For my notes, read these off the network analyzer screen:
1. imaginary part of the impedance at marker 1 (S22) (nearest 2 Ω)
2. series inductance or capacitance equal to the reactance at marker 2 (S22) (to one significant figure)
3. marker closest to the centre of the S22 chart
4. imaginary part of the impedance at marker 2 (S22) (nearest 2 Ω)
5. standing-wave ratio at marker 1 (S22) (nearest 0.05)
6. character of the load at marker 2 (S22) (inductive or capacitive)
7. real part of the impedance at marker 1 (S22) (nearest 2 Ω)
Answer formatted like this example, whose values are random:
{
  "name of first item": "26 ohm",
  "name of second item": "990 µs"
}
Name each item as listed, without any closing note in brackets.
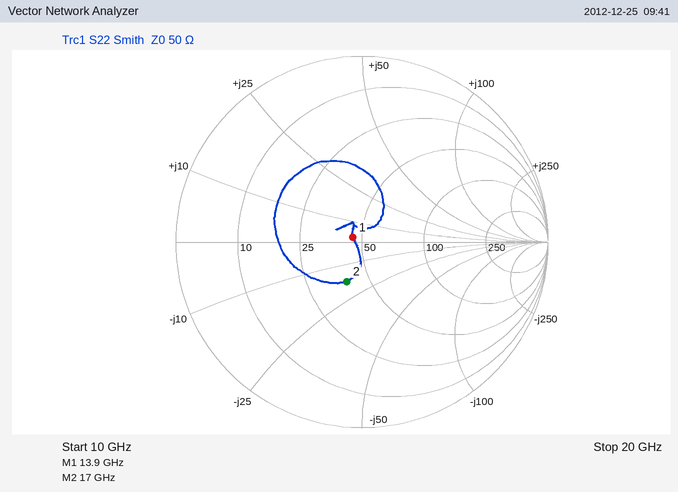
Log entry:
{
  "imaginary part of the impedance at marker 1 (S22)": "+2 Ω",
  "series inductance or capacitance equal to the reactance at marker 2 (S22)": "500 fF",
  "marker closest to the centre of the S22 chart": "marker 1",
  "imaginary part of the impedance at marker 2 (S22)": "-18 Ω",
  "standing-wave ratio at marker 1 (S22)": "1.10",
  "character of the load at marker 2 (S22)": "capacitive",
  "real part of the impedance at marker 1 (S22)": "46 Ω"
}
